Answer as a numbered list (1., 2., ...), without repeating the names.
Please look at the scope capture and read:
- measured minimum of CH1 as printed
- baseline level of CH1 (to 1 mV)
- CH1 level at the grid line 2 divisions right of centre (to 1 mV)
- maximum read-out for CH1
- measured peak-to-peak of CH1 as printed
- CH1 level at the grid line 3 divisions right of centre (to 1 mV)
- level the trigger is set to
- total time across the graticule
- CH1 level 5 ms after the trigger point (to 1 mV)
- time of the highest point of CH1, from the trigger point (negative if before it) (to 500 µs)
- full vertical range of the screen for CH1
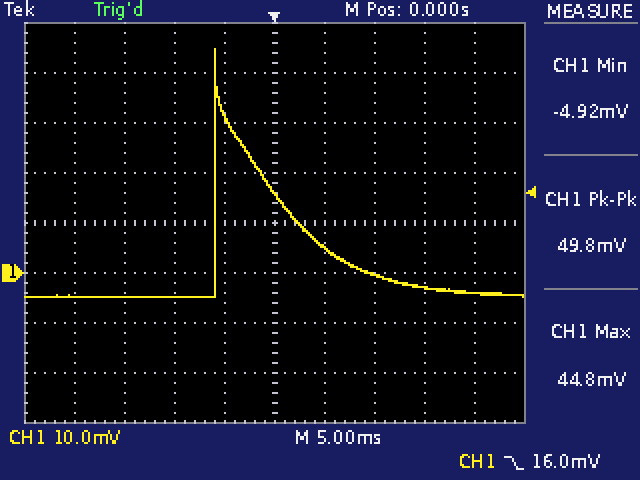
1. -4.92 mV
2. -5 mV
3. 0 mV
4. 44.8 mV
5. 49.8 mV
6. -3 mV
7. 16.0 mV
8. 50 ms
9. 5 mV
10. -6.0 ms
11. 80 mV
